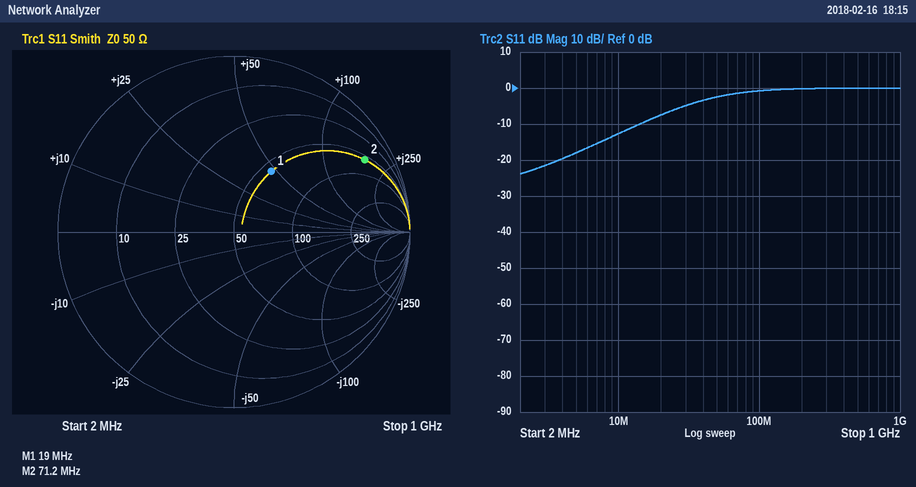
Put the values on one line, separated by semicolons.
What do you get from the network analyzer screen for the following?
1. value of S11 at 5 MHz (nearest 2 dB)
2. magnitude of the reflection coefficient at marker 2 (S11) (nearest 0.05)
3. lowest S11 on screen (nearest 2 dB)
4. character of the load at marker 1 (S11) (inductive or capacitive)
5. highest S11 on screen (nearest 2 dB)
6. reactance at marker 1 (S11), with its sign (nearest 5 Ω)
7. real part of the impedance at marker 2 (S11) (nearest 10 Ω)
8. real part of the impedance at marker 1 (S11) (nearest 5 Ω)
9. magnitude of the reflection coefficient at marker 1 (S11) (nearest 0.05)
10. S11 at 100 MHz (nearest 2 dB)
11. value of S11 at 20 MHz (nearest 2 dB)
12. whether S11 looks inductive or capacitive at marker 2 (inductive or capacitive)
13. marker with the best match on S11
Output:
-18 dB; 0.85; -24 dB; inductive; 0 dB; +45 Ω; 60 Ω; 55 Ω; 0.40; 0 dB; -8 dB; inductive; marker 1
